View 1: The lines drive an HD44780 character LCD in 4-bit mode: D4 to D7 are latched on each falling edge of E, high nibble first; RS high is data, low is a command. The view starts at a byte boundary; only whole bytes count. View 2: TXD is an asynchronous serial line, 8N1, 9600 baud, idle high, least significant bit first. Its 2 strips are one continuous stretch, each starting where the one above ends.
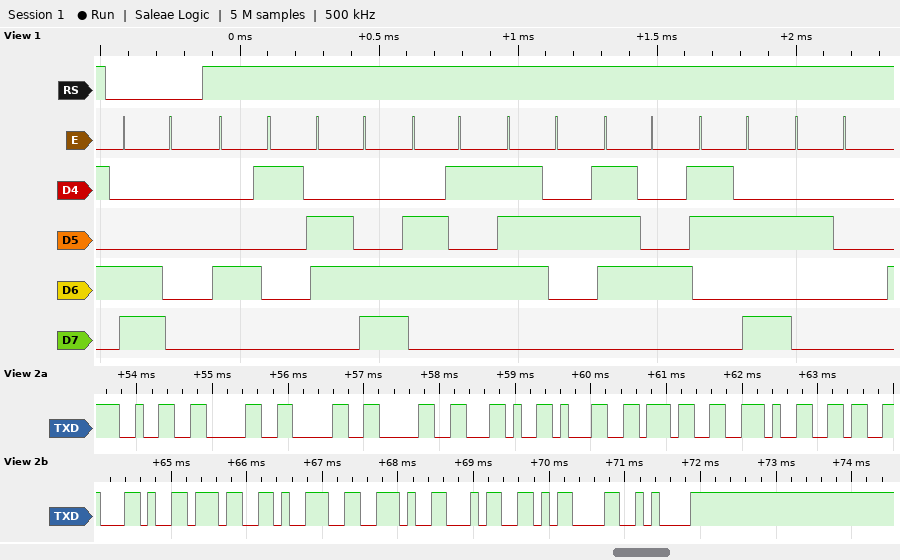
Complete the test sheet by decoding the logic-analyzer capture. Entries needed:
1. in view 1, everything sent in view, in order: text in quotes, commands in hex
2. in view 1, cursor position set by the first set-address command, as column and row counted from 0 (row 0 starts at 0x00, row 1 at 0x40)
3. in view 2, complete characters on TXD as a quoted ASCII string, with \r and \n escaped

0xC0 "Alert: "
column 0, row 1
"2000,17.6,79.4\r\n"
